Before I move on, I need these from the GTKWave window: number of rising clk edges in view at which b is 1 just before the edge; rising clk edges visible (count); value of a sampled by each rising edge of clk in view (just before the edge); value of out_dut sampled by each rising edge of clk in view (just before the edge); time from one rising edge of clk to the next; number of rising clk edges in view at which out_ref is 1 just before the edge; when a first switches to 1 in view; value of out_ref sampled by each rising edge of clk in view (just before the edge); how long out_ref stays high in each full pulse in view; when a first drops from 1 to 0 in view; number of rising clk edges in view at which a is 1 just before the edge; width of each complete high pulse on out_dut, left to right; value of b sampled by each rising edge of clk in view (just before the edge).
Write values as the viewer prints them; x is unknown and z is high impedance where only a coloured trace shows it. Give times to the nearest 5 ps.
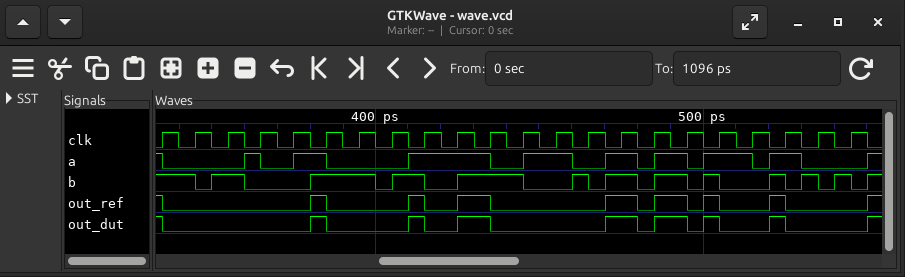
15
22
1 0 0 1 0 1 0 0 1 1 1 0 1 0 1 0 1 1 1 1 0 0
1 0 0 0 0 1 0 0 1 0 1 0 0 0 1 0 1 1 0 1 0 0
10 ps
8
360 ps
1 0 0 0 0 1 0 0 1 0 1 0 0 0 1 0 1 1 0 1 0 0
5 ps, 5 ps, 10 ps, 10 ps, 10 ps, 5 ps, 5 ps
335 ps
12
5 ps, 5 ps, 10 ps, 10 ps, 10 ps, 5 ps, 5 ps
1 1 1 0 0 1 1 0 1 0 1 1 0 1 1 0 1 1 0 1 1 1
